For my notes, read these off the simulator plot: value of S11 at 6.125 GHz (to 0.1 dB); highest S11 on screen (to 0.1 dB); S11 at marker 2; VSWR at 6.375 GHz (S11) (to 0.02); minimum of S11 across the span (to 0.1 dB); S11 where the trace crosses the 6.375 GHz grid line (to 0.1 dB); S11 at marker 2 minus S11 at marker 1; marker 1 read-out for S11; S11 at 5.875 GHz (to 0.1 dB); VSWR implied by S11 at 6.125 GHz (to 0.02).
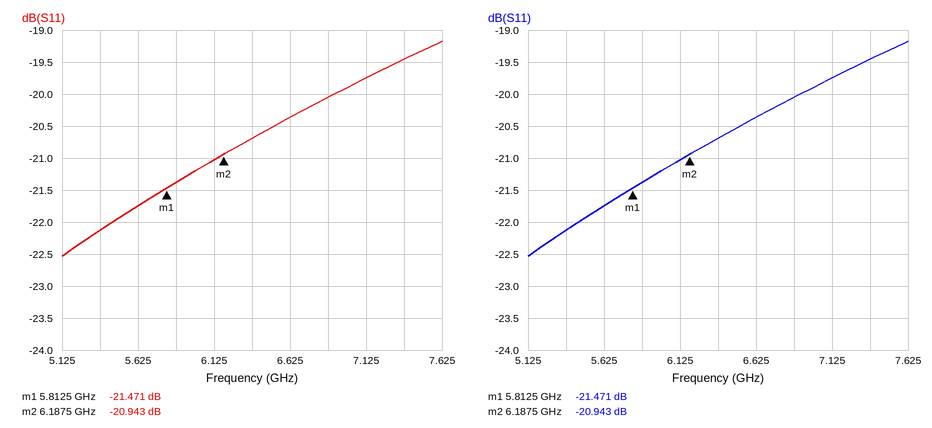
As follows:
-21.0 dB
-19.2 dB
-20.943 dB
1.20
-22.5 dB
-20.7 dB
0.528 dB
-21.471 dB
-21.4 dB
1.20
